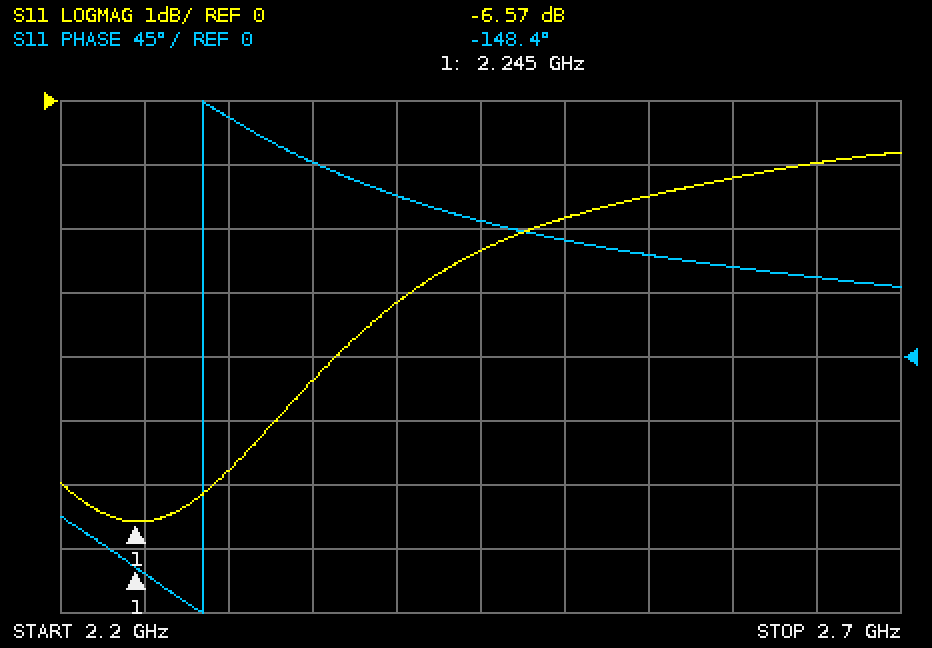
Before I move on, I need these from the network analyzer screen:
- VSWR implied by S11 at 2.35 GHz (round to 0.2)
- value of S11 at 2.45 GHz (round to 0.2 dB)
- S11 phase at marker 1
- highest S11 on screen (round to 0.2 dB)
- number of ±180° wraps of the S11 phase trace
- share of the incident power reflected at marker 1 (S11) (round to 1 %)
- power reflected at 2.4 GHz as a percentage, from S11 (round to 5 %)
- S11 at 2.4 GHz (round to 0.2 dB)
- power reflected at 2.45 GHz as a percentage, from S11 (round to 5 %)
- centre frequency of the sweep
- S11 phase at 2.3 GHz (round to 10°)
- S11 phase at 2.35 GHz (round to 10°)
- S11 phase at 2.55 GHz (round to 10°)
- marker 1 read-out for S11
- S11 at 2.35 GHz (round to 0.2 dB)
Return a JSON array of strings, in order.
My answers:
["4.0", "-2.4 dB", "-148.4°", "-0.8 dB", "1", "22 %", "50 %", "-3.2 dB", "60 %", "2.45 GHz", "170°", "140°", "70°", "-6.57 dB", "-4.4 dB"]
